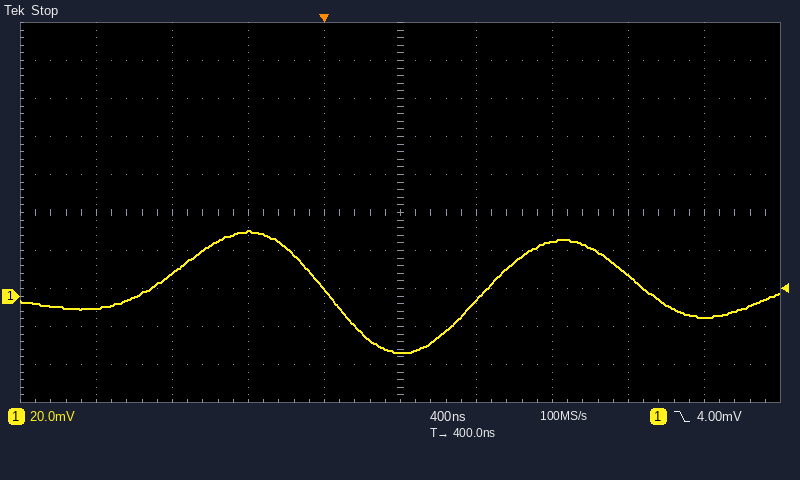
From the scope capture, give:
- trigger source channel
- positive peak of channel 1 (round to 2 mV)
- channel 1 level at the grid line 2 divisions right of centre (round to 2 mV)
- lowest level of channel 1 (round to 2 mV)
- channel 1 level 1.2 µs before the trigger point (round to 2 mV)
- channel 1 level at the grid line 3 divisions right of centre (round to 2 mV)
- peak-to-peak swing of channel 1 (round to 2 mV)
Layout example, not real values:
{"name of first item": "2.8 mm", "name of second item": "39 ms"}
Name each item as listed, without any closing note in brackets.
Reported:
{"trigger source channel": "channel 1", "positive peak of channel 1": "34 mV", "channel 1 level at the grid line 2 divisions right of centre": "28 mV", "lowest level of channel 1": "-30 mV", "channel 1 level 1.2 µs before the trigger point": "-6 mV", "channel 1 level at the grid line 3 divisions right of centre": "12 mV", "peak-to-peak swing of channel 1": "64 mV"}
